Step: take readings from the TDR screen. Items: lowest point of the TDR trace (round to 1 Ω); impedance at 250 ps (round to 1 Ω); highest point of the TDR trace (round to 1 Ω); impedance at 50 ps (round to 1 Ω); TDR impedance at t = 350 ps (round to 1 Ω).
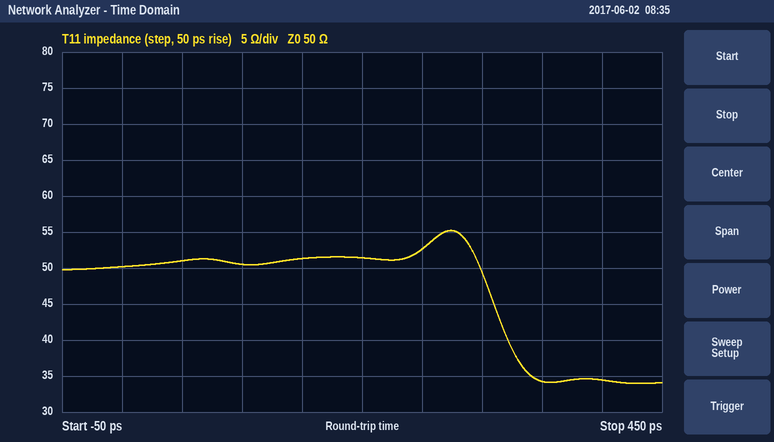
34 Ω
53 Ω
55 Ω
51 Ω
34 Ω
